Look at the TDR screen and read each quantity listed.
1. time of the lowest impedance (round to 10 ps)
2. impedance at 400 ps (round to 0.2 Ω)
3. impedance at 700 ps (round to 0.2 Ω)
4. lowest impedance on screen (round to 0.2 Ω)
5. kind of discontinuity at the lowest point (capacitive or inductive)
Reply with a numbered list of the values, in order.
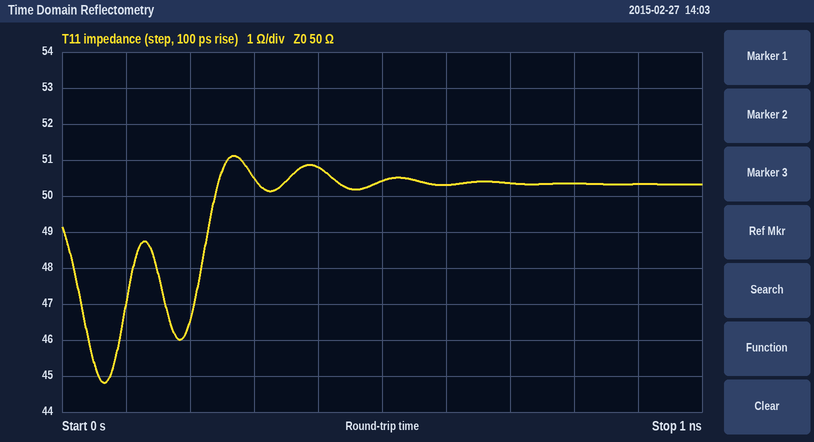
1. 70 ps
2. 50.8 Ω
3. 50.4 Ω
4. 44.8 Ω
5. capacitive
